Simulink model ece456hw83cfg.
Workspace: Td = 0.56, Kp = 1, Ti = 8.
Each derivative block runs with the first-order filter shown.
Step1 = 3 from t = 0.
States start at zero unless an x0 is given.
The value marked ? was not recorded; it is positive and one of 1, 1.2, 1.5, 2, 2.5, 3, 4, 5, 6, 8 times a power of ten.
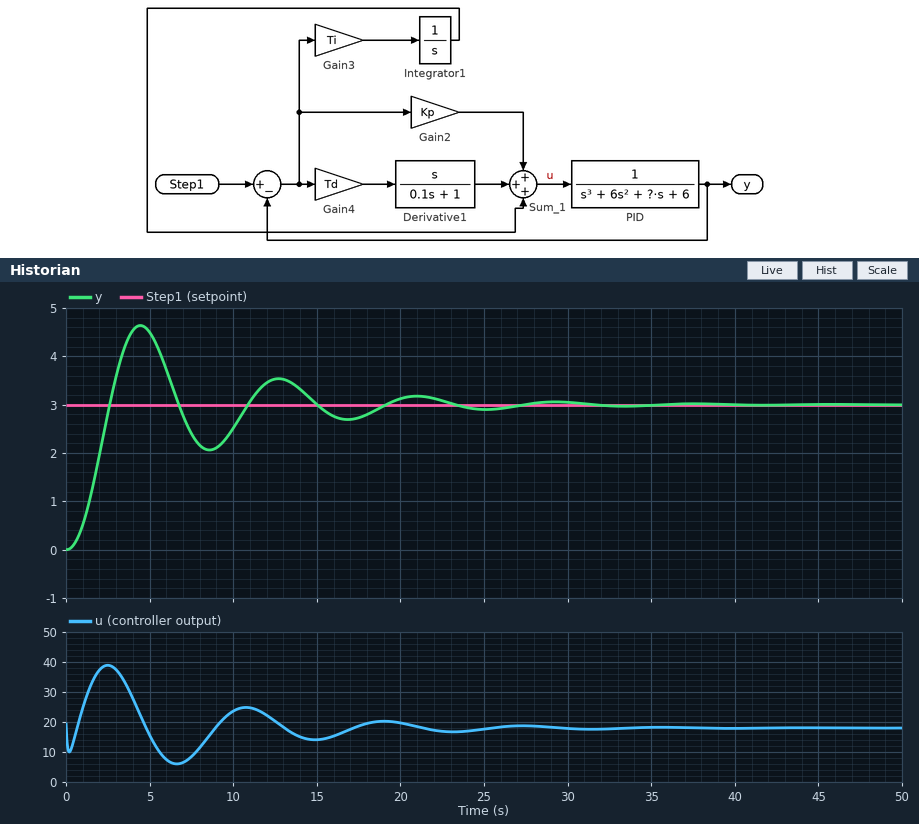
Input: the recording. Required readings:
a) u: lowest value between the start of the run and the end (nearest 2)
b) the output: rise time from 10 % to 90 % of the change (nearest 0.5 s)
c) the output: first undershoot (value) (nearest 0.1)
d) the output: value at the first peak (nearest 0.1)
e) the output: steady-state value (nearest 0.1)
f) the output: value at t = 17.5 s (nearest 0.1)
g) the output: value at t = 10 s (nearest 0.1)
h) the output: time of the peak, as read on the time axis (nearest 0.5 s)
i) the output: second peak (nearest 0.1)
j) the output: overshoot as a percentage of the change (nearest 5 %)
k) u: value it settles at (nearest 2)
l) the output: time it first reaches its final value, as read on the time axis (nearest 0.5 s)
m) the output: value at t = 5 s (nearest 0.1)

6
1.5 s
2.1
4.6
3.0
2.7
2.5
4.5 s
3.5
55 %
18
2.5 s
4.5
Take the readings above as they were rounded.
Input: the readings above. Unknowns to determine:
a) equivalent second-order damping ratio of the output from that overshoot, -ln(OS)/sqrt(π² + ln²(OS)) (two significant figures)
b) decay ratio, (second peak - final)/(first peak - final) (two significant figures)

0.19
0.31
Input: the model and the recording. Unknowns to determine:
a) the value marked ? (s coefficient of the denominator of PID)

15
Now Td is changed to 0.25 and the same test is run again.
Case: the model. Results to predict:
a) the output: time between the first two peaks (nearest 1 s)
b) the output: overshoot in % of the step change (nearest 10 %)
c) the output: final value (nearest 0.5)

8 s
60 %
3.0
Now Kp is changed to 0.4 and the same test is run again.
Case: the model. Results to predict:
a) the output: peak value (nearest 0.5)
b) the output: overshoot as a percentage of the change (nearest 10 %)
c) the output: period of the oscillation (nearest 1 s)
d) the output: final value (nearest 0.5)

5.0
60 %
8 s
3.0
